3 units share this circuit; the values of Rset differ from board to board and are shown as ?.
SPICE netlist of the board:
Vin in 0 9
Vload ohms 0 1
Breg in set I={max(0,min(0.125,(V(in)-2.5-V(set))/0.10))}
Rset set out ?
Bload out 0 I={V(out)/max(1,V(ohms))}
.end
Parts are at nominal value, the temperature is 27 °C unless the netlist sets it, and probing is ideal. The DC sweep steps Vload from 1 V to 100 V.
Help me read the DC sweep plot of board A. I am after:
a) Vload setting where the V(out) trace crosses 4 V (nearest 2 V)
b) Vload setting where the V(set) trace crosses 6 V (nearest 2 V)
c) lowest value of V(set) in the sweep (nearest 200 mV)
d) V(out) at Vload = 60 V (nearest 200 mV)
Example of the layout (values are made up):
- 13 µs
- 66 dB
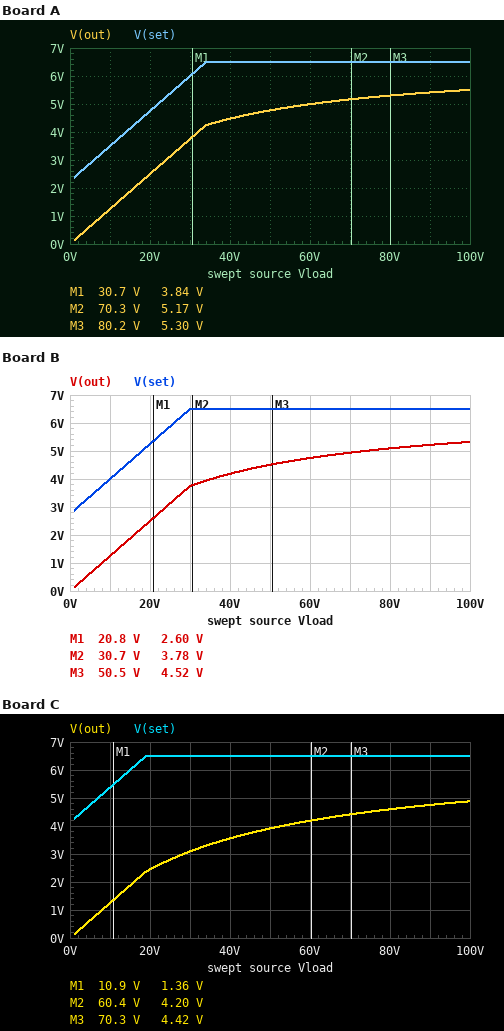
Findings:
- 32 V
- 30 V
- 2.4 V
- 5.0 V
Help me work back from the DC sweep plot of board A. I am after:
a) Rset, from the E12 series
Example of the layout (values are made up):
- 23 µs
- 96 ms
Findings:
- 18 Ω
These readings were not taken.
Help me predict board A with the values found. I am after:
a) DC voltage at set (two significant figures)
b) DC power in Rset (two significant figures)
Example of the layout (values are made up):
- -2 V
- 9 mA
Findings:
- 2.4 V
- 280 mW
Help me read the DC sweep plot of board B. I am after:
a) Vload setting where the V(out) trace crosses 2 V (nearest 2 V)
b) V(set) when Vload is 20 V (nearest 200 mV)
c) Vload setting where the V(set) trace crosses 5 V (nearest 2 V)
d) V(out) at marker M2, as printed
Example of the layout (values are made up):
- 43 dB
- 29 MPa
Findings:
- 16 V
- 5.2 V
- 18 V
- 3.78 V
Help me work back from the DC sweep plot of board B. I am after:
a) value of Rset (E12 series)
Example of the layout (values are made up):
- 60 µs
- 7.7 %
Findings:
- 22 Ω
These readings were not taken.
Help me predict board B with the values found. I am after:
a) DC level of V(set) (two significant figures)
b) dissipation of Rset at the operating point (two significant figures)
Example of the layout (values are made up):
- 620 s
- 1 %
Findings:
- 2.9 V
- 340 mW
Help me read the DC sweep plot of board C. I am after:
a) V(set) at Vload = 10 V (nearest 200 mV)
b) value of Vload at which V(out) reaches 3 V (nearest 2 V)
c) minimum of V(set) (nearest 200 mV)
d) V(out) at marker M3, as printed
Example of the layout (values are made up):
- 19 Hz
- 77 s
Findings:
- 5.4 V
- 28 V
- 4.2 V
- 4.42 V
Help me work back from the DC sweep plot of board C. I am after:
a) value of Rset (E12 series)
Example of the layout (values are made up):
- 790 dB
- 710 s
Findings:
- 33 Ω
